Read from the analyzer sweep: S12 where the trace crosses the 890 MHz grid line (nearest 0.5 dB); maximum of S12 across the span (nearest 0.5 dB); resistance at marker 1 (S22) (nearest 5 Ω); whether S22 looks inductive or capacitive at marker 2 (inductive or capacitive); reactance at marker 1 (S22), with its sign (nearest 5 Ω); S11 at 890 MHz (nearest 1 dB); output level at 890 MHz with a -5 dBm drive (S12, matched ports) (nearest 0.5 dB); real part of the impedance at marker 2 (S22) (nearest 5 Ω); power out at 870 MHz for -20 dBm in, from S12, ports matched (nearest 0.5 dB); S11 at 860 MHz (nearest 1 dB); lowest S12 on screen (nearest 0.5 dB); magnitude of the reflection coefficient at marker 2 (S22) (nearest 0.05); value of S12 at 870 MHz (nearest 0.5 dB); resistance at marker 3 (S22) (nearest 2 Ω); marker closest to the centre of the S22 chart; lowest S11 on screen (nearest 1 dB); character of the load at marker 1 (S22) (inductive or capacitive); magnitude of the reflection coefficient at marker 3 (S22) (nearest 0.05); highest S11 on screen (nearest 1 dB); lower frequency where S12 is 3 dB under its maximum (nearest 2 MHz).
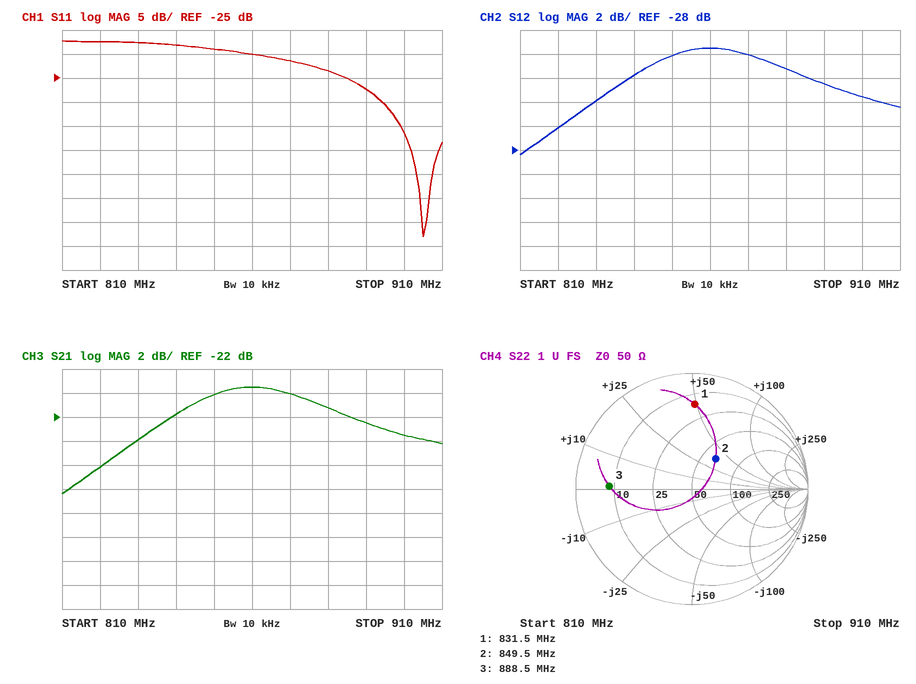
-22.5 dB
-19.5 dB
15 Ω
inductive
+50 Ω
-27 dB
-27.5 dBm
65 Ω
-40.0 dBm
-20 dB
-28.5 dB
0.35
-20.0 dB
8 Ω
marker 2
-58 dB
inductive
0.70
-17 dB
836 MHz
